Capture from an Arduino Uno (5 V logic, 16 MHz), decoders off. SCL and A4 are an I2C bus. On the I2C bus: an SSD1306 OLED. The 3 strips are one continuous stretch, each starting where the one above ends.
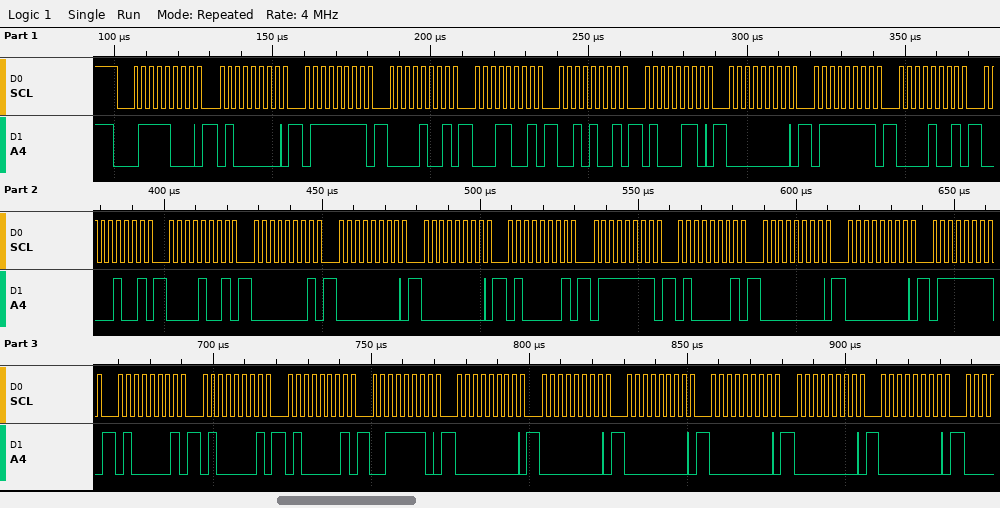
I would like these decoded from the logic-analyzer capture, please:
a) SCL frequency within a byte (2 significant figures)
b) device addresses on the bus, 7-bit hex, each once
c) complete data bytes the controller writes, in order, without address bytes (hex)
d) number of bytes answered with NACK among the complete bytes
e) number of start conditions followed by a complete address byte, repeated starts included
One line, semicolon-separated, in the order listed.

400 kHz; 0x3C; 40 7F 09 19 29 46 00 7F 09 09 09 01 00 00 41 7F 41 00 00 7F 41 41 41 3E 00 00 00 00 00 00; 0; 1
